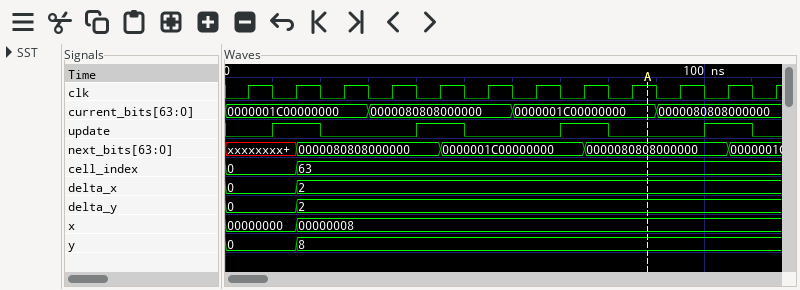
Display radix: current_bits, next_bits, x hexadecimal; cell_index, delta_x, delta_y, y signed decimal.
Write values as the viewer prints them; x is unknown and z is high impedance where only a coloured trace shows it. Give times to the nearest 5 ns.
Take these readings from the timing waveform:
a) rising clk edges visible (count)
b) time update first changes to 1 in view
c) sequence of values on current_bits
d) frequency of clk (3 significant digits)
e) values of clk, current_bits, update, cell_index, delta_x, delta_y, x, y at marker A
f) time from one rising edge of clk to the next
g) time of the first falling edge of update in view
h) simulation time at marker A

12
10 ns
0000001C00000000, 0000080808000000, 0000001C00000000, 0000080808000000
100 MHz
clk=1, current_bits=0000001C00000000, update=0, cell_index=63, delta_x=2, delta_y=2, x=00000008, y=8
10 ns
20 ns
90 ns
